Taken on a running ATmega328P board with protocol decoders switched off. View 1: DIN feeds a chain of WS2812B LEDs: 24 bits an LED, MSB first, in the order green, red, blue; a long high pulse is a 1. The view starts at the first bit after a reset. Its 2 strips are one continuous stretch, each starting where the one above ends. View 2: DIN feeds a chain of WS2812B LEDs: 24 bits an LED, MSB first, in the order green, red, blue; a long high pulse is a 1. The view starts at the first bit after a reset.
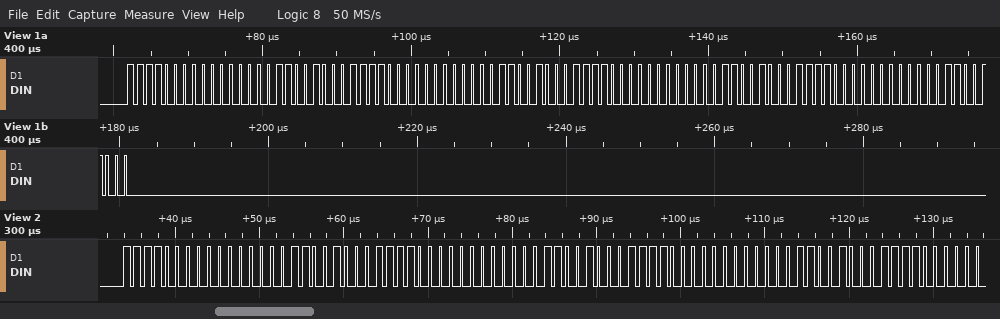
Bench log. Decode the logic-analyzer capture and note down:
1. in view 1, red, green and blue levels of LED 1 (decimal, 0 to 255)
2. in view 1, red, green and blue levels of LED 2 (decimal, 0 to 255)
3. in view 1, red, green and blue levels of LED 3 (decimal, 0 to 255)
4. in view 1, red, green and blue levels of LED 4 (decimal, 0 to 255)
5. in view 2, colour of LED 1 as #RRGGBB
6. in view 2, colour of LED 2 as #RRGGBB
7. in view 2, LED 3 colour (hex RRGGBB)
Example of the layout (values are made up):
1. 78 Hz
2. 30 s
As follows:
1. 0, 240, 200
2. 0, 240, 200
3. 0, 240, 200
4. 0, 240, 200
5. #00F0C8
6. #00F0C8
7. #00F0C8
